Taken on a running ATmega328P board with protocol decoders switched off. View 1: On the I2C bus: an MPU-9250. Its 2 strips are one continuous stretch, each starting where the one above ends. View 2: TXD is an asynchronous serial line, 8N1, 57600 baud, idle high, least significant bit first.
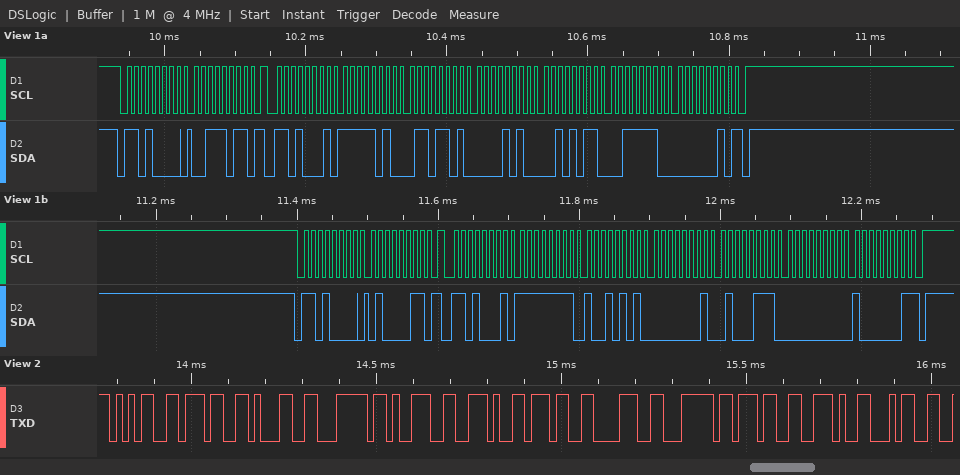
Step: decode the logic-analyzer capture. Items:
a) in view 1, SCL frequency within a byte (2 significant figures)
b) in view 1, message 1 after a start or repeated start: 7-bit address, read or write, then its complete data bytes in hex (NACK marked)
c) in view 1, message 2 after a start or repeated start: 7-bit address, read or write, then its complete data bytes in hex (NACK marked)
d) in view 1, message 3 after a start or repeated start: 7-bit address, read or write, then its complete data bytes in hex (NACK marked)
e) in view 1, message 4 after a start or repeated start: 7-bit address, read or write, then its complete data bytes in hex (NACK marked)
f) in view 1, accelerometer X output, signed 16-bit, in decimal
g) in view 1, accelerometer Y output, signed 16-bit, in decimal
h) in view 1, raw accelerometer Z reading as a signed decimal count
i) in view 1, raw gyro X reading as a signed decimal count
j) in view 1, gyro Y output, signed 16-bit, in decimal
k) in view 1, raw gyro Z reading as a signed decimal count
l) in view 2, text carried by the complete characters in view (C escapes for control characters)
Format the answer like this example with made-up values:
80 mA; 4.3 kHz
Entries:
100 kHz; 0x68 write: 3B; 0x68 read: FA 6D 0A 2B 3E 02 NACK; 0x68 write: 43; 0x68 read: FF 95 01 47 00 81 NACK; -1427; 2603; 15874; -107; 327; 129; "571|9.78|7.4"
